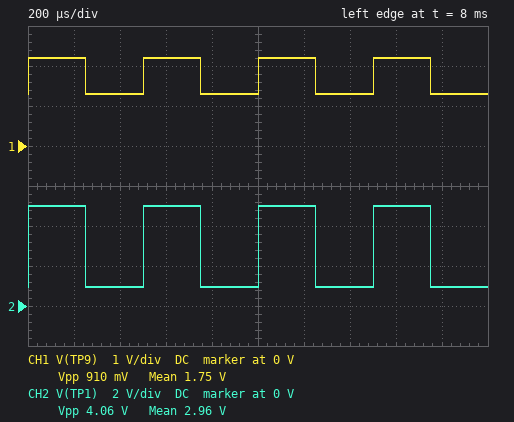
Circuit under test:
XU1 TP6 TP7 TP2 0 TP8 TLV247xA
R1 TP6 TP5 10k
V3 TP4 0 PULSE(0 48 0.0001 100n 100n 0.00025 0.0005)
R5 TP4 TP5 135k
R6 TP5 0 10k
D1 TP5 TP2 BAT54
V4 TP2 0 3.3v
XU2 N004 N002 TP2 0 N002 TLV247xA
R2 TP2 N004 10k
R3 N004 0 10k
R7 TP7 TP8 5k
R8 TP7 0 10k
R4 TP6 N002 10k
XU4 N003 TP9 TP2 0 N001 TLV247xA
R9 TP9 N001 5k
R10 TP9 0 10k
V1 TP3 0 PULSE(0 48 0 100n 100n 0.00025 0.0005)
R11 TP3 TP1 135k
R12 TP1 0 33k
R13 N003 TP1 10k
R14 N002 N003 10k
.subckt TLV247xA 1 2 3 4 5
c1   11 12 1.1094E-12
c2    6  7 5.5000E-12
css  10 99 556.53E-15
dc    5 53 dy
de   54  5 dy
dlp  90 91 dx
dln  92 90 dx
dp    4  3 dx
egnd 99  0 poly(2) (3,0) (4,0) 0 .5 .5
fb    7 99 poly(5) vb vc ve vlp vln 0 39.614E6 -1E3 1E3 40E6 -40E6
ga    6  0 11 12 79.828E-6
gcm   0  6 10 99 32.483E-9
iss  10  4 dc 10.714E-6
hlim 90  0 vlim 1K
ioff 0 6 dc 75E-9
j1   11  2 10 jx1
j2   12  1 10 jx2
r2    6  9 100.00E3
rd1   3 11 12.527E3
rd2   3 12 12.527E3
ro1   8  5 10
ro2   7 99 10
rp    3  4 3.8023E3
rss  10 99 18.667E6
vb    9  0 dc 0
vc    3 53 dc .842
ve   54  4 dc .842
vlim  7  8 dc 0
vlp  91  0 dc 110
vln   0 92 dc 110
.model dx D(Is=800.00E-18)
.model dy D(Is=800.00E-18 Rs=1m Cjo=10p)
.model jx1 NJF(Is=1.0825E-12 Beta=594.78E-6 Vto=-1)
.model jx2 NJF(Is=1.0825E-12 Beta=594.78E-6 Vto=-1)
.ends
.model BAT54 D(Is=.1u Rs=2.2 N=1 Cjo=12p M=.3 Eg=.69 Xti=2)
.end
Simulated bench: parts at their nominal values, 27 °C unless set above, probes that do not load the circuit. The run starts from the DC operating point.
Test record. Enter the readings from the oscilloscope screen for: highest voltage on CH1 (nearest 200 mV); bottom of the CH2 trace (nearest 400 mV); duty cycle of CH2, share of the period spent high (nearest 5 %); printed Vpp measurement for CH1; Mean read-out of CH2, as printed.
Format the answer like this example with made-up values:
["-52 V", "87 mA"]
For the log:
["2.2 V", "800 mV", "50 %", "910 mV", "2.96 V"]
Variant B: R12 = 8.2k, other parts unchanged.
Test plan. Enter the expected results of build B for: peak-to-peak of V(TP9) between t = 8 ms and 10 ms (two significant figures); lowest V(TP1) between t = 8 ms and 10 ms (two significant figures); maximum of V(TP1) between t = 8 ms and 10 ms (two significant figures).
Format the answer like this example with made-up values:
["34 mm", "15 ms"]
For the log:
["990 mV", "460 mV", "2.4 V"]
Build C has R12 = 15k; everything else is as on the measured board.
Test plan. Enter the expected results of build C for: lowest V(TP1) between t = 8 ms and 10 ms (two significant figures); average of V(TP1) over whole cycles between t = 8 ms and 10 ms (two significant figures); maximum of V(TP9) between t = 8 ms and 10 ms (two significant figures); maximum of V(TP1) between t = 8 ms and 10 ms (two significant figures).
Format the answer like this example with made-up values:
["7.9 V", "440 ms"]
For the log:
["660 mV", "2.1 V", "2.2 V", "3.5 V"]
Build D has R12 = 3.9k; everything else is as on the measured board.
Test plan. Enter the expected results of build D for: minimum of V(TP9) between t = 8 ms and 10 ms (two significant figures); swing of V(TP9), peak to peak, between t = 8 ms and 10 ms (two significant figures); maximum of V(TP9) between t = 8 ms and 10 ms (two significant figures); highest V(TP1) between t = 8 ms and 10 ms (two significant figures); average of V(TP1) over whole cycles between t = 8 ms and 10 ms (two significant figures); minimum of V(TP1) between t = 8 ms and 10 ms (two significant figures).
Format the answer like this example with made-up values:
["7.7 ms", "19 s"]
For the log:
["950 mV", "570 mV", "1.5 V", "1.4 V", "830 mV", "260 mV"]
